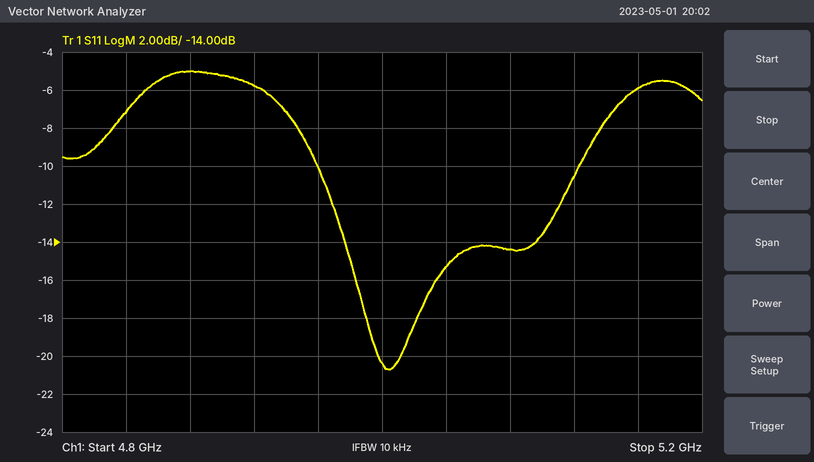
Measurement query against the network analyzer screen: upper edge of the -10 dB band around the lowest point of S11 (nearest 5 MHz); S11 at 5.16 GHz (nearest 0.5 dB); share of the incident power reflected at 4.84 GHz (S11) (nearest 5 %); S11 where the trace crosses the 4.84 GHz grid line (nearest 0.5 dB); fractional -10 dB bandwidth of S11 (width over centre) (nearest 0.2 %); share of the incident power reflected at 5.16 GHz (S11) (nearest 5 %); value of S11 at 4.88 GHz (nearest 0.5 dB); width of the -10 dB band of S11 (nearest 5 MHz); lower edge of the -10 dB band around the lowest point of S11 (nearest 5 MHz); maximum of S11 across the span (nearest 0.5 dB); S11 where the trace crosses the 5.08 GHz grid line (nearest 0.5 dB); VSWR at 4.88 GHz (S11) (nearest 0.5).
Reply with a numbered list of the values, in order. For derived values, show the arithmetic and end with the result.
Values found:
1. 5.125 GHz
2. -6.0 dB
3. 10^(-7/10) ≈ 20 %
4. -7.0 dB
5. 165 MHz / 5.0425 GHz ≈ 3.27 %, so 3.2 % to the nearest 0.2 %
6. 10^(-6/10) ≈ 25 %
7. -5.0 dB
8. 5.125 GHz − 4.960 GHz = 165 MHz
9. 4.960 GHz
10. -5.0 dB
11. -14.5 dB
12. |Γ| = 10^(-5/20) = 0.5623; VSWR = (1 + 0.5623)/(1 − 0.5623) ≈ 3.57, so 3.5 to the nearest 0.5
